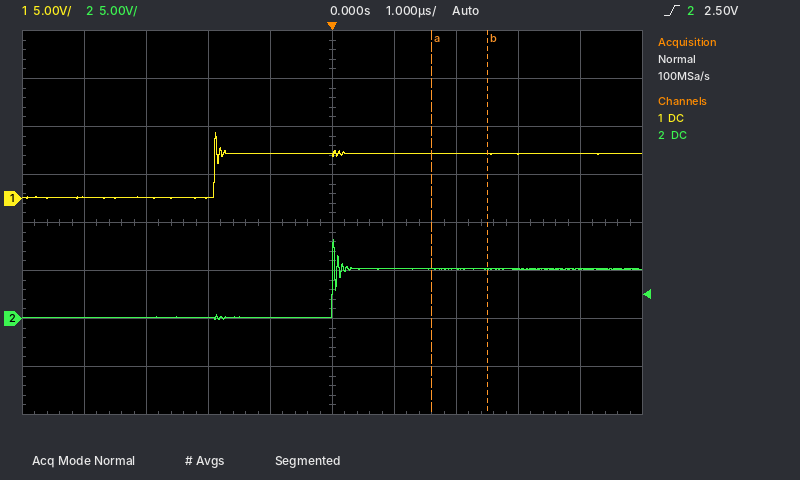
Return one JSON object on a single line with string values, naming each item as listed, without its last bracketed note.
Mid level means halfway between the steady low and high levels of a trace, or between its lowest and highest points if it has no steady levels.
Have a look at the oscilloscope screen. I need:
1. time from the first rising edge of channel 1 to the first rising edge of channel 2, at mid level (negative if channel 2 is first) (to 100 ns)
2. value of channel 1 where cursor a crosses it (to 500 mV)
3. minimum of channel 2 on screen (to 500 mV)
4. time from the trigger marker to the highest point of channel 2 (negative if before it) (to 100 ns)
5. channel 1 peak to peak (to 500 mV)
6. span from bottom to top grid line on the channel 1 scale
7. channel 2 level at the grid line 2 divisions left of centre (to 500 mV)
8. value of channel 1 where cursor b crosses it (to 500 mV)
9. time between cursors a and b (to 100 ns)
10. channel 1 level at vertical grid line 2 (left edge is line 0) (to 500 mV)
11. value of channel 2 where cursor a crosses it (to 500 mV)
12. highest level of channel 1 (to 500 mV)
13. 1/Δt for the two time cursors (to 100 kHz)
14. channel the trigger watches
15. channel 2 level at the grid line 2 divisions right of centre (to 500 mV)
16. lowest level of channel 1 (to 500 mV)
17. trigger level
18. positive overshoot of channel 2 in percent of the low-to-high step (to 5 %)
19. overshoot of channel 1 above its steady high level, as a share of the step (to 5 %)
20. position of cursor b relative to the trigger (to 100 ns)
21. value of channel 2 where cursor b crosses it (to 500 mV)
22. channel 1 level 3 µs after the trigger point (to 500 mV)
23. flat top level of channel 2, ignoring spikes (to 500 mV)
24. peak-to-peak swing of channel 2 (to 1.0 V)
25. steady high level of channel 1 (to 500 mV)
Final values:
{"time from the first rising edge of channel 1 to the first rising edge of channel 2, at mid level (negative if channel 2 is first)": "+1.9 µs", "value of channel 1 where cursor a crosses it": "4.5 V", "minimum of channel 2 on screen": "0.0 V", "time from the trigger marker to the highest point of channel 2 (negative if before it)": "0.0 µs", "channel 1 peak to peak": "7.0 V", "span from bottom to top grid line on the channel 1 scale": "40 V", "channel 2 level at the grid line 2 divisions left of centre": "0.0 V", "value of channel 1 where cursor b crosses it": "4.5 V", "time between cursors a and b": "900 ns", "channel 1 level at vertical grid line 2 (left edge is line 0)": "0.0 V", "value of channel 2 where cursor a crosses it": "5.0 V", "highest level of channel 1": "7.0 V", "1/Δt for the two time cursors": "1.1 MHz", "channel the trigger watches": "channel 2", "channel 2 level at the grid line 2 divisions right of centre": "5.0 V", "lowest level of channel 1": "0.0 V", "trigger level": "2.50 V", "positive overshoot of channel 2 in percent of the low-to-high step": "60 %", "overshoot of channel 1 above its steady high level, as a share of the step": "50 %", "position of cursor b relative to the trigger": "+2.5 µs", "value of channel 2 where cursor b crosses it": "5.0 V", "channel 1 level 3 µs after the trigger point": "4.5 V", "flat top level of channel 2, ignoring spikes": "5.0 V", "peak-to-peak swing of channel 2": "8.0 V", "steady high level of channel 1": "4.5 V"}
